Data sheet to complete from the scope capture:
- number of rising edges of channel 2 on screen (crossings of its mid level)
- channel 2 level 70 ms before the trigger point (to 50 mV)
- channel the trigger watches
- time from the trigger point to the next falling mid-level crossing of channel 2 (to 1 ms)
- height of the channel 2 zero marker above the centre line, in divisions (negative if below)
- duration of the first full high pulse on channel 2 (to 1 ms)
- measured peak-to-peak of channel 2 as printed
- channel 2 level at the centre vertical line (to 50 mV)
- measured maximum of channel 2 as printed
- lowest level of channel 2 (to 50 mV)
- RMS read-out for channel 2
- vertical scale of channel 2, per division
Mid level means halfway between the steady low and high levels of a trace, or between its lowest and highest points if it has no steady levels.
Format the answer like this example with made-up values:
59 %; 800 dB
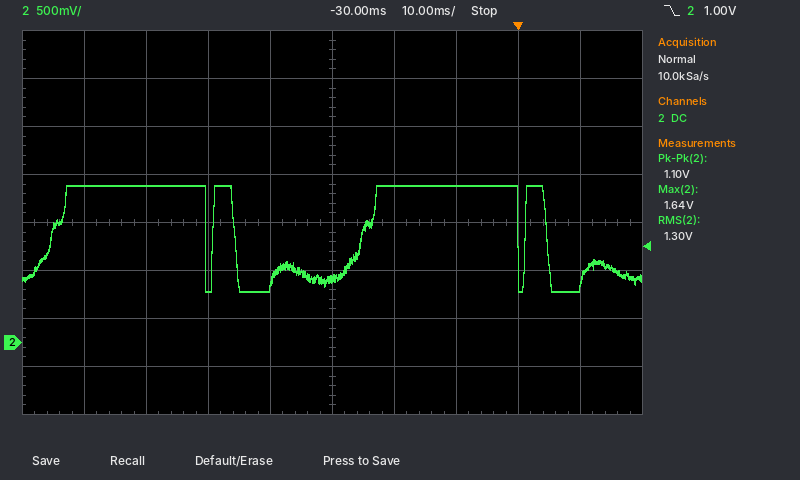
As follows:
4; 1.65 V; channel 2; 5 ms; -2.5 div; 25 ms; 1.10 V; 650 mV; 1.64 V; 550 mV; 1.30 V; 500 mV
